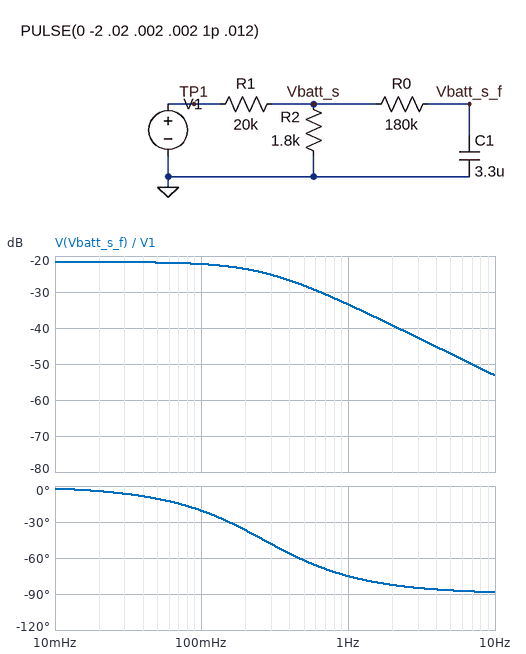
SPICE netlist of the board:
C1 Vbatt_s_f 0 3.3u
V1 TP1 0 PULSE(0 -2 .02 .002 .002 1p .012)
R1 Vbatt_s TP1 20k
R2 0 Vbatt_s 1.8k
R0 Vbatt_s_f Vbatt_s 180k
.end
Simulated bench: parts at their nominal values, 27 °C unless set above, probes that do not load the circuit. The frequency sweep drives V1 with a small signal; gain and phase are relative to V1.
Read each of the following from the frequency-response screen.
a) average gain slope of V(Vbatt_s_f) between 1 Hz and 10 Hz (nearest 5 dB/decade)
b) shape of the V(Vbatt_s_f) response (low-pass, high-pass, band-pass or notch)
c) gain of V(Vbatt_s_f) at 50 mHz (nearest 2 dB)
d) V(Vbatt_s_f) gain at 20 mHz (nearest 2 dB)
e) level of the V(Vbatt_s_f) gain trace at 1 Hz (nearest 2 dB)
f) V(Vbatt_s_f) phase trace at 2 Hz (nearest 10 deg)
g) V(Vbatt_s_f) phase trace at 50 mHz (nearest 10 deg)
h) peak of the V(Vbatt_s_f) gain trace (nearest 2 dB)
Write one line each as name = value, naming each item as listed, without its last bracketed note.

average gain slope of V(Vbatt_s_f) between 1 Hz and 10 Hz = -20 dB/decade
shape of the V(Vbatt_s_f) response = low-pass
gain of V(Vbatt_s_f) at 50 mHz = -22 dB
V(Vbatt_s_f) gain at 20 mHz = -22 dB
level of the V(Vbatt_s_f) gain trace at 1 Hz = -34 dB
V(Vbatt_s_f) phase trace at 2 Hz = -80 deg
V(Vbatt_s_f) phase trace at 50 mHz = -10 deg
peak of the V(Vbatt_s_f) gain trace = -22 dB
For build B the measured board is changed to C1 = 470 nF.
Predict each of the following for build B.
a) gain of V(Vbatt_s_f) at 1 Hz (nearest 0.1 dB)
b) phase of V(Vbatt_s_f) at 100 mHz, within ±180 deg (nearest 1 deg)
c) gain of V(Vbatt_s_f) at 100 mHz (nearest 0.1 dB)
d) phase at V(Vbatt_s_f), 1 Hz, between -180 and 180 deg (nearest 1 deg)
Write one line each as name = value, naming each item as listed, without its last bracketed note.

gain of V(Vbatt_s_f) at 1 Hz = -22.8 dB
phase of V(Vbatt_s_f) at 100 mHz, within ±180 deg = -3 deg
gain of V(Vbatt_s_f) at 100 mHz = -21.7 dB
phase at V(Vbatt_s_f), 1 Hz, between -180 and 180 deg = -28 deg
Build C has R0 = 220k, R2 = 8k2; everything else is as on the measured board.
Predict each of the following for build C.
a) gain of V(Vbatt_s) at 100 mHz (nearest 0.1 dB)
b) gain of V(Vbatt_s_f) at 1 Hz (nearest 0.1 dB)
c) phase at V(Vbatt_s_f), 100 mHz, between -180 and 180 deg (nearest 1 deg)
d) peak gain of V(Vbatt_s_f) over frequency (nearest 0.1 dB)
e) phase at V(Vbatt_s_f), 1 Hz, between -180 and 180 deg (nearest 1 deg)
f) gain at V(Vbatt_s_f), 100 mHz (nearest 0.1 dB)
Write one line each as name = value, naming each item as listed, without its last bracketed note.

gain of V(Vbatt_s) at 100 mHz = -10.8 dB
gain of V(Vbatt_s_f) at 1 Hz = -24.3 dB
phase at V(Vbatt_s_f), 100 mHz, between -180 and 180 deg = -25 deg
peak gain of V(Vbatt_s_f) over frequency = -10.7 dB
phase at V(Vbatt_s_f), 1 Hz, between -180 and 180 deg = -78 deg
gain at V(Vbatt_s_f), 100 mHz = -11.6 dB
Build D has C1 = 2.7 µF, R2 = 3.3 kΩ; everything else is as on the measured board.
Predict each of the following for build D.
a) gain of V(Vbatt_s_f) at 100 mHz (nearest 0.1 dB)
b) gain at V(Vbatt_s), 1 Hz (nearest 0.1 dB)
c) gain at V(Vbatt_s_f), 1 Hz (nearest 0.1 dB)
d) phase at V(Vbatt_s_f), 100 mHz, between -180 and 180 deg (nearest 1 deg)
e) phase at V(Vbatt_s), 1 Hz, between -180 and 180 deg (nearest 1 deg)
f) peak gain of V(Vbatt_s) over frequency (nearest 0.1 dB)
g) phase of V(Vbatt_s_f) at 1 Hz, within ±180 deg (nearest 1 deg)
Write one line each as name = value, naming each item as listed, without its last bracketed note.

gain of V(Vbatt_s_f) at 100 mHz = -17.4 dB
gain at V(Vbatt_s), 1 Hz = -17.1 dB
gain at V(Vbatt_s_f), 1 Hz = -27.2 dB
phase at V(Vbatt_s_f), 100 mHz, between -180 and 180 deg = -17 deg
phase at V(Vbatt_s), 1 Hz, between -180 and 180 deg = 0 deg
peak gain of V(Vbatt_s) over frequency = -17.0 dB
phase of V(Vbatt_s_f) at 1 Hz, within ±180 deg = -72 deg
